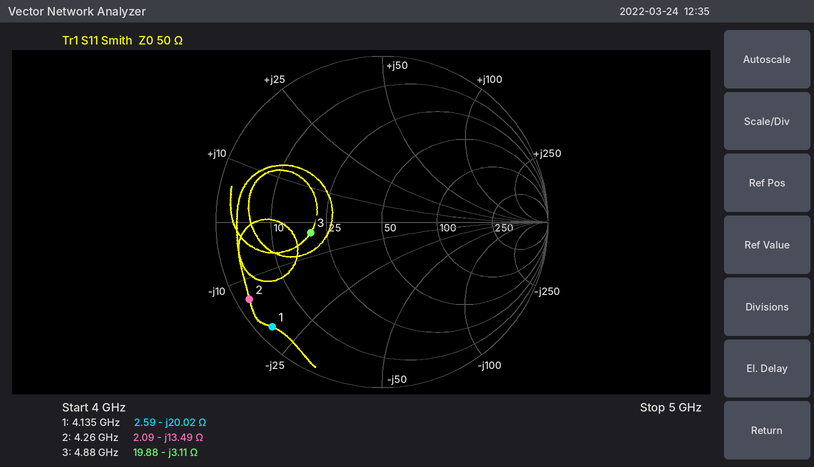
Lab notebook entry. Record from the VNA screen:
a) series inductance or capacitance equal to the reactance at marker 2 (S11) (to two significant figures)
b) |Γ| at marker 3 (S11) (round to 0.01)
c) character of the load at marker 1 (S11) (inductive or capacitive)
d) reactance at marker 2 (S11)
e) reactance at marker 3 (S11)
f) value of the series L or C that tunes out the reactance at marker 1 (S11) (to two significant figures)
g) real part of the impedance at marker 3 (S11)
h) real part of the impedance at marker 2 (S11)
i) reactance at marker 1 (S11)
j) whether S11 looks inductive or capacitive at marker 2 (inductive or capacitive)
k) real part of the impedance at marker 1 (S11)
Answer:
2.8 pF
0.43
capacitive
-13.49 Ω
-3.11 Ω
770 pH
19.88 Ω
2.09 Ω
-20.02 Ω
capacitive
2.59 Ω
